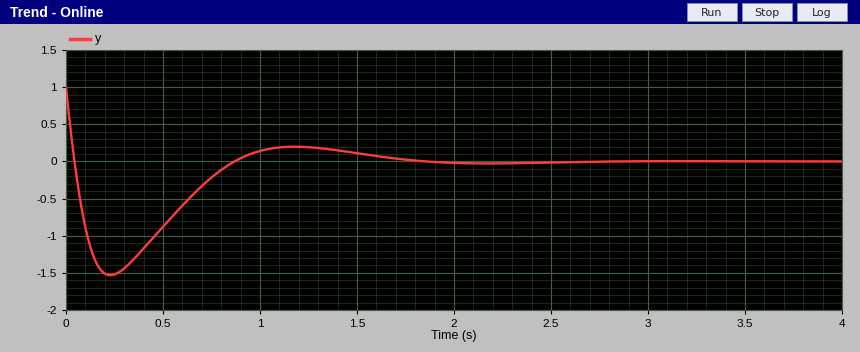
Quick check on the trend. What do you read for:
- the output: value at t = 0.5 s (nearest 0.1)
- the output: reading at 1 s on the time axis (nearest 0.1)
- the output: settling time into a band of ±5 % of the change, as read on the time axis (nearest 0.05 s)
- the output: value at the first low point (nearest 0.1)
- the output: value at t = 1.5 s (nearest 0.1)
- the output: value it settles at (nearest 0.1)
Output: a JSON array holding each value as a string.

["-0.9", "0.1", "1.65 s", "-1.5", "0.1", "0.0"]
